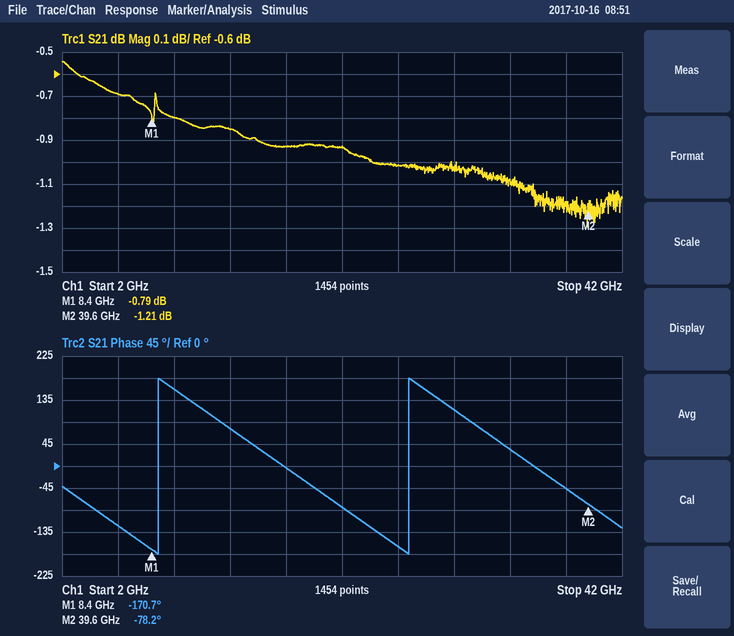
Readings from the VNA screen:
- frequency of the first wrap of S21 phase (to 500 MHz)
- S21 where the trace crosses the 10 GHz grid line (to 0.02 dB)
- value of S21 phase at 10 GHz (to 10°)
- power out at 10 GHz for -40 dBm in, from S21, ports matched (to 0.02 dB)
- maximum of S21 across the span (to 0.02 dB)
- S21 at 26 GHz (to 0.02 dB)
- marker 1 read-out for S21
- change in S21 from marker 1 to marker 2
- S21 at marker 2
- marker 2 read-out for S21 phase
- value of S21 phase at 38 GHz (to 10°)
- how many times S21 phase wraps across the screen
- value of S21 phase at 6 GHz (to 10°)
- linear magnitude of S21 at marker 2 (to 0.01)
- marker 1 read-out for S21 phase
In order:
9.0 GHz
-0.80 dB
160°
-40.80 dBm
-0.54 dB
-1.02 dB
-0.79 dB
-0.42 dB
-1.21 dB
-78.2°
-50°
2
-120°
0.87
-170.7°
